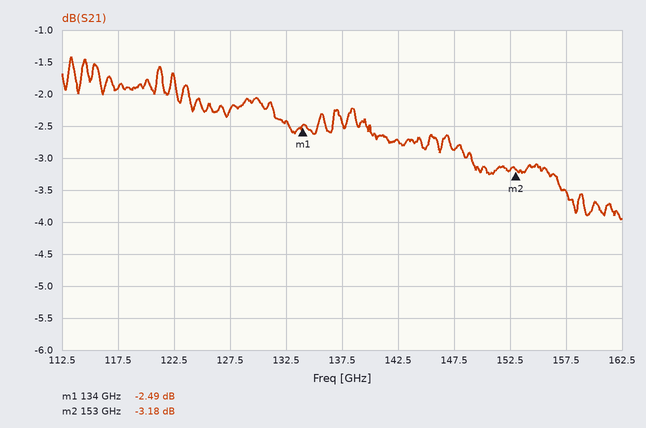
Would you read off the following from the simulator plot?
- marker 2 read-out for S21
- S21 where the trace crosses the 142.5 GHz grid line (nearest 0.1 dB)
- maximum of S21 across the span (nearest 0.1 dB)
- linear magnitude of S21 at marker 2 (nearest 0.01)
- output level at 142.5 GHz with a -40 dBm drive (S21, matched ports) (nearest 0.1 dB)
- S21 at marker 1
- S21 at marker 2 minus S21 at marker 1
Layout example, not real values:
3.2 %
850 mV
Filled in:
-3.18 dB
-2.7 dB
-1.4 dB
0.69
-42.7 dBm
-2.49 dB
-0.69 dB
